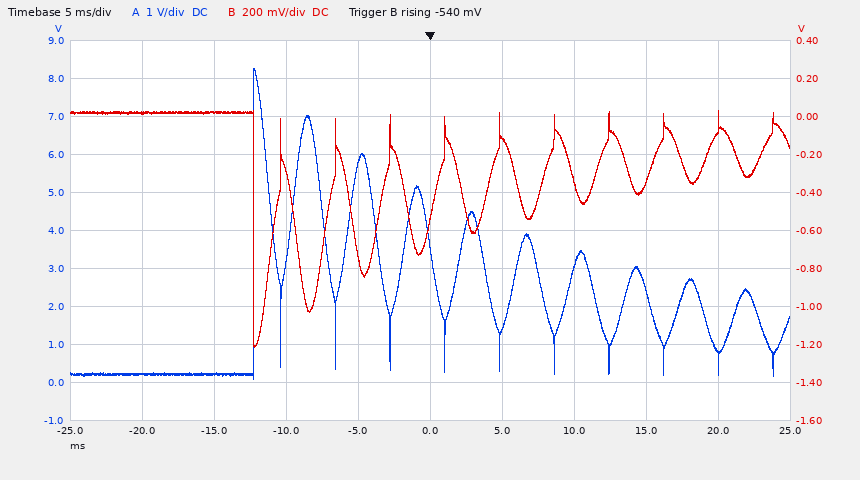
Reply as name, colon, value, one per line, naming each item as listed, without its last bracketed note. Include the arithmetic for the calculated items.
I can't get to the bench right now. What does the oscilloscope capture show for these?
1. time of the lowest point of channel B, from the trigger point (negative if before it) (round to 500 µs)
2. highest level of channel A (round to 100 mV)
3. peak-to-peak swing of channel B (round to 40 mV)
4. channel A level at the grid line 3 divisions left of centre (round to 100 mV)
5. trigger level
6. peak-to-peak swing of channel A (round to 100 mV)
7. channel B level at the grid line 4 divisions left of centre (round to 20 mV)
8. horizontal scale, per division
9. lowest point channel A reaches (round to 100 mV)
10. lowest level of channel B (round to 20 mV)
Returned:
time of the lowest point of channel B, from the trigger point (negative if before it): -12.0 ms
highest level of channel A: 8.3 V
peak-to-peak swing of channel B: 1.24 V
channel A level at the grid line 3 divisions left of centre: 200 mV
trigger level: -540 mV
peak-to-peak swing of channel A: 8.3 V − (100 mV) = 8.2 V
channel B level at the grid line 4 divisions left of centre: 20 mV
horizontal scale, per division: 5 ms
lowest point channel A reaches: 100 mV
lowest level of channel B: -1.22 V
